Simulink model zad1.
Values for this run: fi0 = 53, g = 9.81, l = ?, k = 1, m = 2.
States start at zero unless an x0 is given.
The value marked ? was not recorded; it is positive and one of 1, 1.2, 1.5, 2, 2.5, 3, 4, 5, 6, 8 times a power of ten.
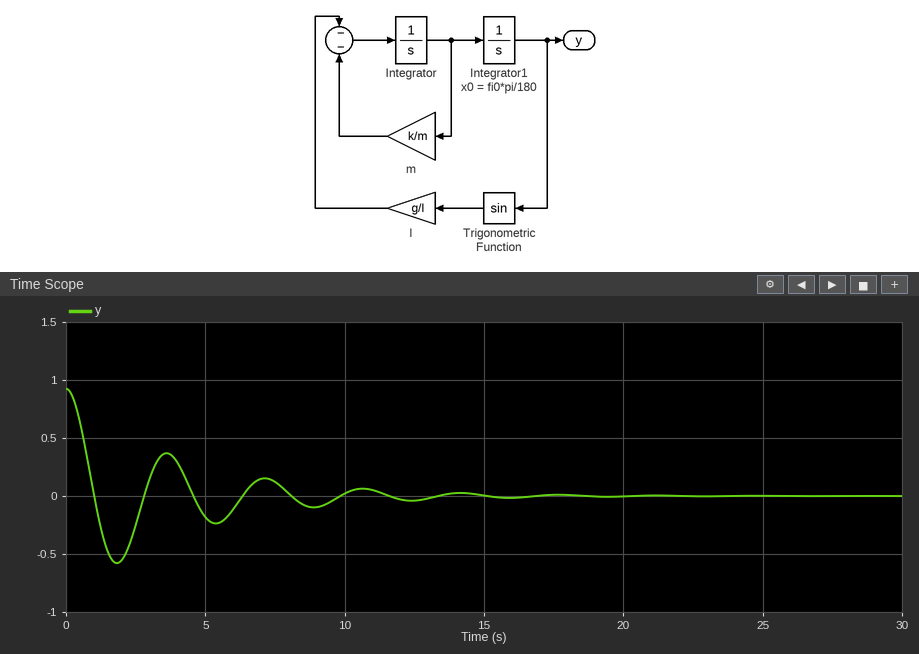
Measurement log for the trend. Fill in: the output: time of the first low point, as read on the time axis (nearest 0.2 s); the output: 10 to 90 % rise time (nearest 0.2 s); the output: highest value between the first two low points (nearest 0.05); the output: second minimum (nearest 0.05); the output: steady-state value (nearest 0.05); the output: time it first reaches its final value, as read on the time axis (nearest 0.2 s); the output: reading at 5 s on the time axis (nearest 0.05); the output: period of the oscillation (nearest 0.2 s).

1.8 s
0.6 s
0.35
-0.25
0.00
1.0 s
-0.20
3.6 s
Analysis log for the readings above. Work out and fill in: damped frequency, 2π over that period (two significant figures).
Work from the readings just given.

1.7 rad/s
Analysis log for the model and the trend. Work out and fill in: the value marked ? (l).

3
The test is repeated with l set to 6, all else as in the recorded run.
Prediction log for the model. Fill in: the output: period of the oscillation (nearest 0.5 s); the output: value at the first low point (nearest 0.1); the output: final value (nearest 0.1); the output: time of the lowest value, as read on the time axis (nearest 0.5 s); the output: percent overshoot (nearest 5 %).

5.0 s
-0.5
0.0
2.5 s
50 %
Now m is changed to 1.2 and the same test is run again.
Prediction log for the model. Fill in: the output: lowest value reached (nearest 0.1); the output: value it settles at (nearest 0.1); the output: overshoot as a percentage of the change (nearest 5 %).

-0.4
0.0
45 %
